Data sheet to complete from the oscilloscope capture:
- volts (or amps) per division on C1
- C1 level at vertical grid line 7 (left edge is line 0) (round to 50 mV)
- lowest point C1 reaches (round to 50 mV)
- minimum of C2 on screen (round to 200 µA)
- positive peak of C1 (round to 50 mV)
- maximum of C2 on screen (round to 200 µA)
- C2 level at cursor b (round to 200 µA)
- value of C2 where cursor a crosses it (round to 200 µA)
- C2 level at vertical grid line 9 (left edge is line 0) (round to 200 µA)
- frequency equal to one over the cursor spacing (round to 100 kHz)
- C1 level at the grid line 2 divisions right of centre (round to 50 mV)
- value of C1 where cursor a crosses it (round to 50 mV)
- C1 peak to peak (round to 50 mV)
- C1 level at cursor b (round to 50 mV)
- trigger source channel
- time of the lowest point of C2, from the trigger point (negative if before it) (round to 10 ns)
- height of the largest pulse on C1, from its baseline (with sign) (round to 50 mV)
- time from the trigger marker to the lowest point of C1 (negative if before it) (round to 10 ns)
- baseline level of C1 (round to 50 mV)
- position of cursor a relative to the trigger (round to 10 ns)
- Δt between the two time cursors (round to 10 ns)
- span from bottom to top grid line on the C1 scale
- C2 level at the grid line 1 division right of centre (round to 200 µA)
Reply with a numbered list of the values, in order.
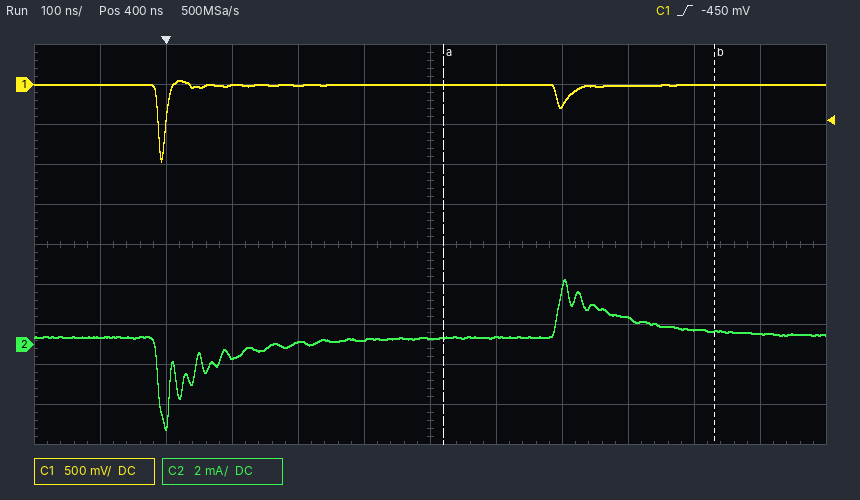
1. 500 mV
2. 0 mV
3. -950 mV
4. -4.2 mA
5. 50 mV
6. 3.2 mA
7. 600 µA
8. 400 µA
9. 1.4 mA
10. 2.4 MHz
11. -250 mV
12. 0 mV
13. 1.00 V
14. 0 mV
15. C1
16. 0 ns
17. -950 mV
18. -10 ns
19. 0 mV
20. +420 ns
21. 410 ns
22. 5 V
23. 400 µA
